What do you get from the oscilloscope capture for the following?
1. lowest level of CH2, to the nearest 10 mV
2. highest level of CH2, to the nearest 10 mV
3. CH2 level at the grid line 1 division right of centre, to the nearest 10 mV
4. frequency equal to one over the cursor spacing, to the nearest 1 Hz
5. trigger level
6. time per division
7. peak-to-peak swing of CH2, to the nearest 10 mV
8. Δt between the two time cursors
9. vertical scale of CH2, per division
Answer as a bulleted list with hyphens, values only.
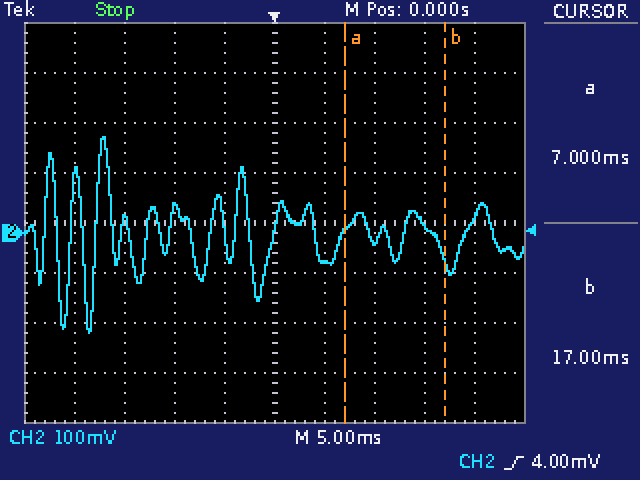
- -200 mV
- 190 mV
- -60 mV
- 100 Hz
- 4.00 mV
- 5 ms
- 390 mV
- 10.0 ms
- 100 mV
